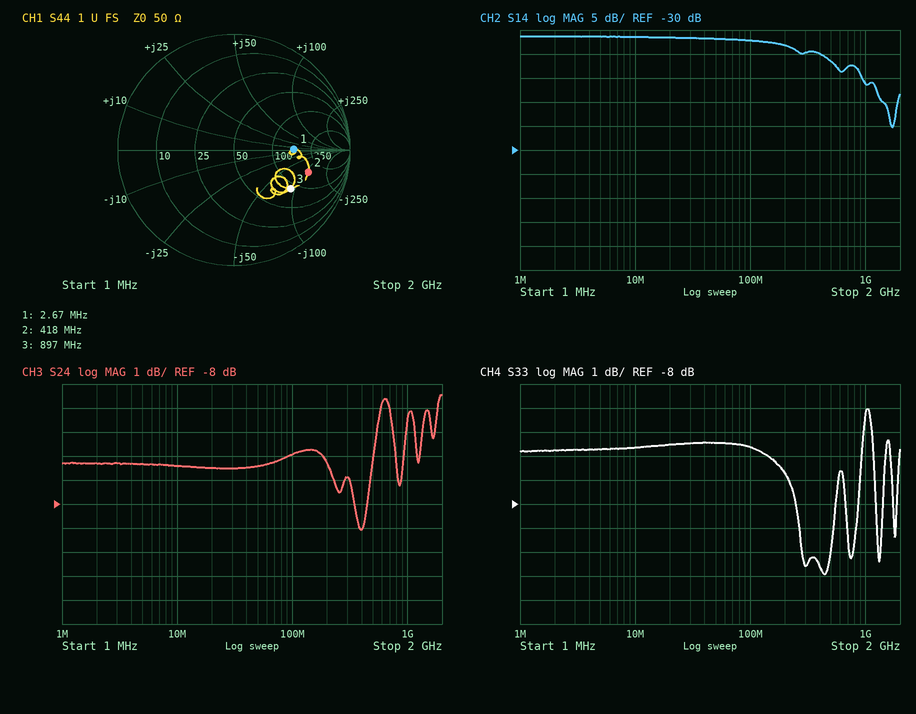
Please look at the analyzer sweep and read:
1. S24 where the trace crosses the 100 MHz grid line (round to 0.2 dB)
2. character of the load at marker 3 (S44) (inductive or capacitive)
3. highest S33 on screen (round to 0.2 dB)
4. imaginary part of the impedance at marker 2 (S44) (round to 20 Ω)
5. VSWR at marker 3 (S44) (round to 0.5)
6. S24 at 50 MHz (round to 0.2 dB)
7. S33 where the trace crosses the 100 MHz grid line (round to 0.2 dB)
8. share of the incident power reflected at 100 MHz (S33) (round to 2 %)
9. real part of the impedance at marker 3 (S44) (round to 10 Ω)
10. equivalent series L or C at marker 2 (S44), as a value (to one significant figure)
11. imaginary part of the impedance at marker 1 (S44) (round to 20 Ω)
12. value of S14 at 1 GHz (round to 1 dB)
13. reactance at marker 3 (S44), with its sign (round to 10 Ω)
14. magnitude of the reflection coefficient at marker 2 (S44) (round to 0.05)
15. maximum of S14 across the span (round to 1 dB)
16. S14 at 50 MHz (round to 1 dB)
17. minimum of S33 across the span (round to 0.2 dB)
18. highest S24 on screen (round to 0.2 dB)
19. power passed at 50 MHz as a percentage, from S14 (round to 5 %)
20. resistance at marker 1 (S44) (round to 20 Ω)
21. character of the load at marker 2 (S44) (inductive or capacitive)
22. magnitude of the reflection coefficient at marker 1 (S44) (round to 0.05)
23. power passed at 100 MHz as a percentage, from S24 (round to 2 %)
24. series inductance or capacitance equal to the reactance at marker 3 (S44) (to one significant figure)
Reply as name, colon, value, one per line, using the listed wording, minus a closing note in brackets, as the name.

S24 where the trace crosses the 100 MHz grid line: -6.0 dB
character of the load at marker 3 (S44): capacitive
highest S33 on screen: -4.0 dB
imaginary part of the impedance at marker 2 (S44): -120 Ω
VSWR at marker 3 (S44): 4.0
S24 at 50 MHz: -6.4 dB
S33 where the trace crosses the 100 MHz grid line: -5.6 dB
share of the incident power reflected at 100 MHz (S33): 28 %
real part of the impedance at marker 3 (S44): 90 Ω
equivalent series L or C at marker 2 (S44), as a value: 3 pF
imaginary part of the impedance at marker 1 (S44): 0 Ω
value of S14 at 1 GHz: -16 dB
reactance at marker 3 (S44), with its sign: -90 Ω
magnitude of the reflection coefficient at marker 2 (S44): 0.65
maximum of S14 across the span: -6 dB
S14 at 50 MHz: -7 dB
minimum of S33 across the span: -11.0 dB
highest S24 on screen: -3.4 dB
power passed at 50 MHz as a percentage, from S14: 20 %
resistance at marker 1 (S44): 160 Ω
character of the load at marker 2 (S44): capacitive
magnitude of the reflection coefficient at marker 1 (S44): 0.50
power passed at 100 MHz as a percentage, from S24: 26 %
series inductance or capacitance equal to the reactance at marker 3 (S44): 2 pF
